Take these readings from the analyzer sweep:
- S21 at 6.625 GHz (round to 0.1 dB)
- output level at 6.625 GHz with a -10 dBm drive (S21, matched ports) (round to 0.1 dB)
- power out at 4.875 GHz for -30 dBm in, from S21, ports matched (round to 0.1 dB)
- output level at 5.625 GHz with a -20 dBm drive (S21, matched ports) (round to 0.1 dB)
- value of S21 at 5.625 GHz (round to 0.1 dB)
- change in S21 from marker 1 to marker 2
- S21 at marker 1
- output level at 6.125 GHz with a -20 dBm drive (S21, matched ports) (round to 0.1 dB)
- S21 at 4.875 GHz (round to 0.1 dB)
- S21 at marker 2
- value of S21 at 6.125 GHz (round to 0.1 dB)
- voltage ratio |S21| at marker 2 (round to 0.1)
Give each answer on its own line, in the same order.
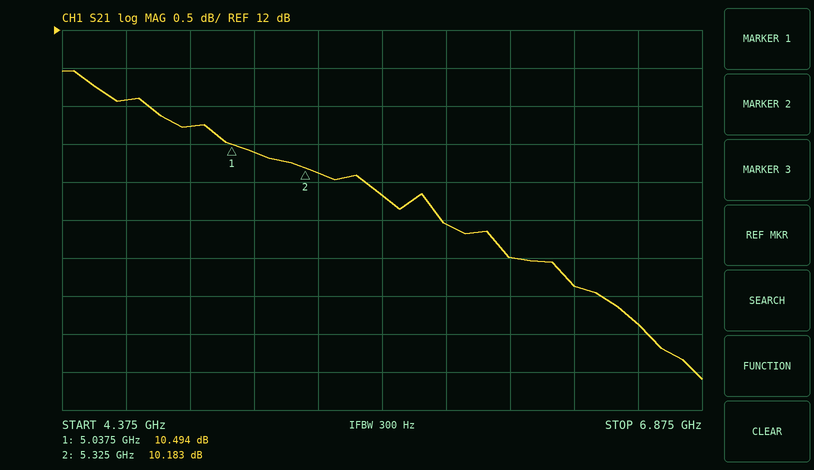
8.1 dB
-1.9 dBm
-19.3 dBm
-10.2 dBm
9.8 dB
-0.311 dB
10.494 dB
-11.0 dBm
10.7 dB
10.183 dB
9.0 dB
3.2
